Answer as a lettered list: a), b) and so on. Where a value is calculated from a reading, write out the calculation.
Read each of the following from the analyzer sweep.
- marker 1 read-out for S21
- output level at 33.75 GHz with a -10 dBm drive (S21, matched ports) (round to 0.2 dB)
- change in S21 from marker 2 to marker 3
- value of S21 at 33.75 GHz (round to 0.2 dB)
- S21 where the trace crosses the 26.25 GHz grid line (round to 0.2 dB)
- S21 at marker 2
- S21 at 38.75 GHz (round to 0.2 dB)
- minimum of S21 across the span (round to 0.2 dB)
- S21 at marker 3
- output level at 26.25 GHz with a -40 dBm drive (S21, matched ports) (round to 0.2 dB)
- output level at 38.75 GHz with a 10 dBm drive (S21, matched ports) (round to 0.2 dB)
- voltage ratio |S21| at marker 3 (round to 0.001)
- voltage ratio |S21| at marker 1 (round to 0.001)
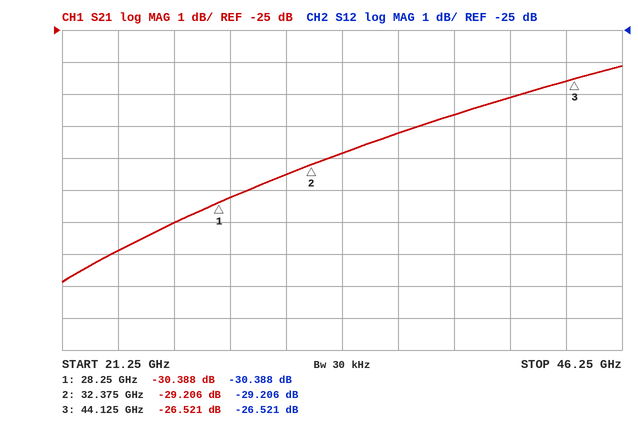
a) -30.388 dB
b) -10 dBm + (-28.8 dB) = -38.8 dBm
c) -26.521 − (-29.206) = 2.685 dB
d) -28.8 dB
e) -31.0 dB
f) -29.206 dB
g) -27.6 dB
h) -32.8 dB
i) -26.521 dB
j) -40 dBm + (-31.0 dB) = -71.0 dBm
k) 10 dBm + (-27.6 dB) = -17.6 dBm
l) 10^(-26.521/20) ≈ 0.047
m) 10^(-30.388/20) ≈ 0.030
